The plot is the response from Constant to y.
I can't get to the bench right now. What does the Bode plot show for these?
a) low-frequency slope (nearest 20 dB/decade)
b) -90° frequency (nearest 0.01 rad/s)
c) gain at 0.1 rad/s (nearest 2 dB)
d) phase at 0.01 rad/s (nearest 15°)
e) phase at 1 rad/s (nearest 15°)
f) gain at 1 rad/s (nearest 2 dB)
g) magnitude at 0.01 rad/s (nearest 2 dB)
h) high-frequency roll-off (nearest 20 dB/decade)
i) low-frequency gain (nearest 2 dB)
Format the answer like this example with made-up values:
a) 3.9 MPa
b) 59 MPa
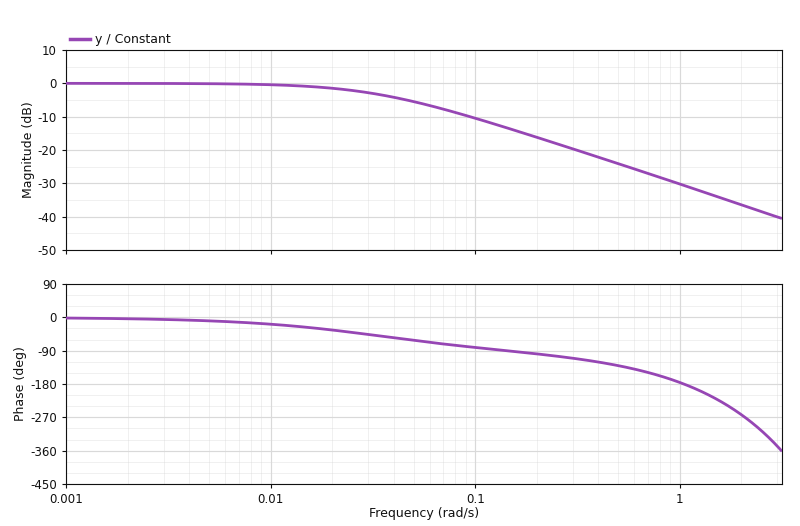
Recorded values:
a) 0 dB/decade
b) 0.14 rad/s
c) -10 dB
d) -15°
e) -180°
f) -30 dB
g) 0 dB
h) -20 dB/decade
i) 0 dB
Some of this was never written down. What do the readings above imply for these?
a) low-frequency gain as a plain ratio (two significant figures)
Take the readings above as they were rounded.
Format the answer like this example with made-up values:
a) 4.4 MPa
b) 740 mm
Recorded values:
a) 1.0
